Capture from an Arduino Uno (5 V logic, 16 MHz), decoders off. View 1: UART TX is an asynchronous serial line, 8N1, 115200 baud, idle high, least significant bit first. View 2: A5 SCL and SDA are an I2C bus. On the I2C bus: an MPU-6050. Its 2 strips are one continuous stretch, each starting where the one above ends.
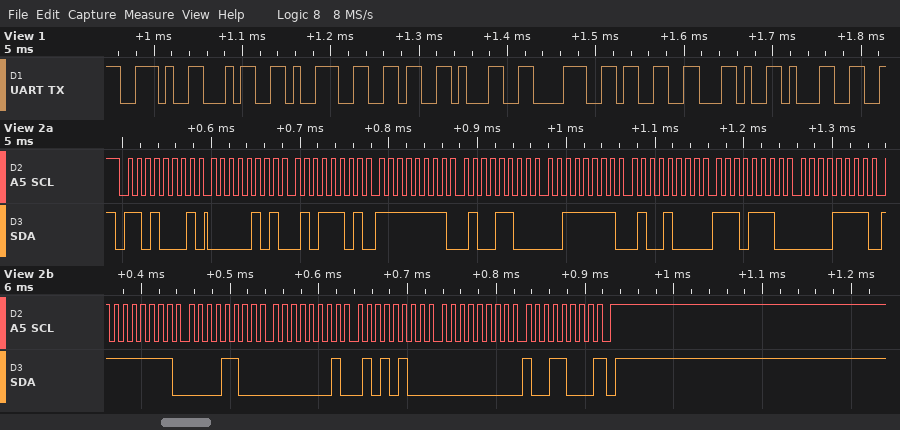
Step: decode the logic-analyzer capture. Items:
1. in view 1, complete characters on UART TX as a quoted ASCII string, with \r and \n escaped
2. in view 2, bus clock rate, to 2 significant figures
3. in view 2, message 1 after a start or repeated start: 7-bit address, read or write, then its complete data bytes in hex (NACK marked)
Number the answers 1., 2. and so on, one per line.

1. ".496183,1"
2. 100 kHz
3. 0x68 read: 05 5D FF 4C 3F 48 EE 0F FF 0C 01 54 00 98 NACK
